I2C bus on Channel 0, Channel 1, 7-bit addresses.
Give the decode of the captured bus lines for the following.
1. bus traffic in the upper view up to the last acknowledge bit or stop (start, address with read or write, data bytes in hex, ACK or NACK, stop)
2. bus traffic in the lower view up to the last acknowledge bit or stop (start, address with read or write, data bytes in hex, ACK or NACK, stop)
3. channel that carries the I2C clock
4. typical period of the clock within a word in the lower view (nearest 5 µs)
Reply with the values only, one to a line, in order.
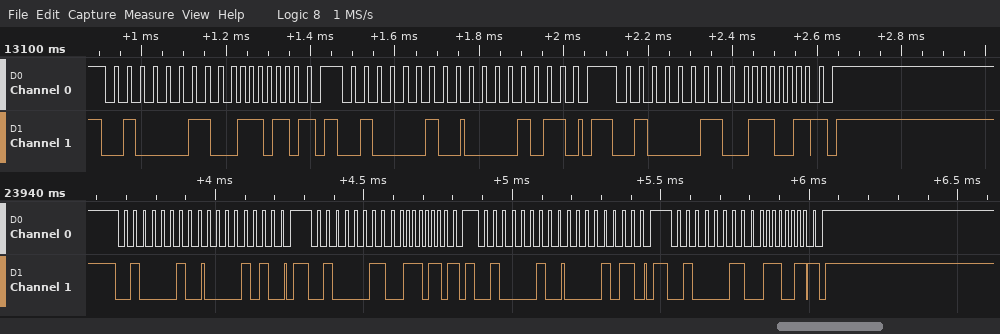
start, address 21 read ACK, 76 NACK, stop, start, address 21 write ACK, 0B ACK, stop, start, address 21 read ACK, 73 NACK, stop
start, address 21 write ACK, 0A ACK, stop, start, address 21 read ACK, 76 NACK, stop, start, address 21 write ACK, 0B ACK, stop, start, address 21 read ACK, 73 NACK, stop
Channel 0
30 µs
